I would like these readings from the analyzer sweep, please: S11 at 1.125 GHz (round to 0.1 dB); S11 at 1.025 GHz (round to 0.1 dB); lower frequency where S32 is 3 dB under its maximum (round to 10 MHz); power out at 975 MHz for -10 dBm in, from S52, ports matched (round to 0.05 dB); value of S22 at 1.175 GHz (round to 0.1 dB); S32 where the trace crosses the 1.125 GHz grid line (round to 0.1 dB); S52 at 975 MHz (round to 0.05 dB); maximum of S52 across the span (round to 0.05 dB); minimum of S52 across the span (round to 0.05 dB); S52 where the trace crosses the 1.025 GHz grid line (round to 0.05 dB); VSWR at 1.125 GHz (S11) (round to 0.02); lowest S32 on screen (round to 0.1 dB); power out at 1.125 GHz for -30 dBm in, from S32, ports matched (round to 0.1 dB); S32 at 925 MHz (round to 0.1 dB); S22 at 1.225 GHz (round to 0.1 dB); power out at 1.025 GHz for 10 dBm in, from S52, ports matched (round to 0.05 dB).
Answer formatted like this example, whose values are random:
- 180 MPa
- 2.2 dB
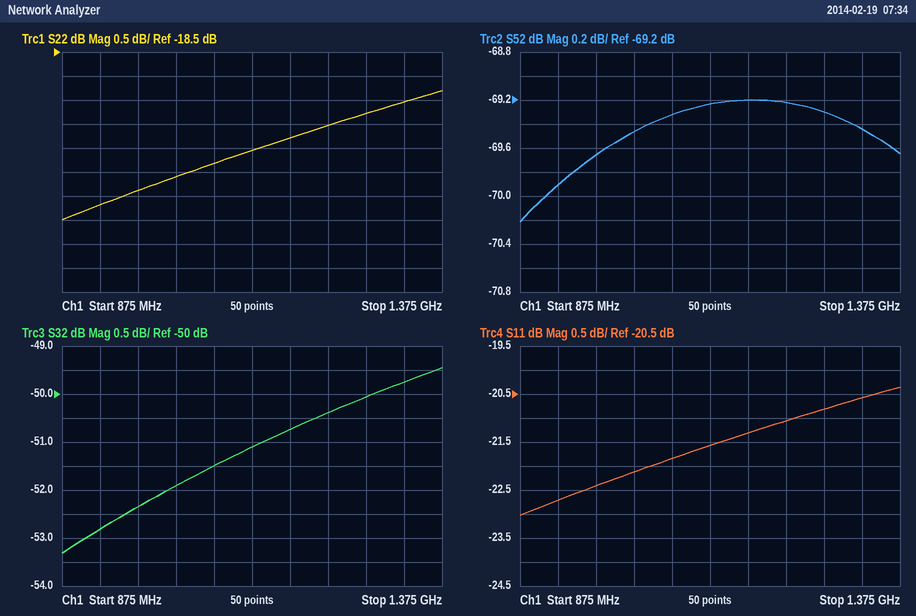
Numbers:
- -21.6 dB
- -22.1 dB
- 960 MHz
- -79.65 dBm
- -20.3 dB
- -51.1 dB
- -69.65 dB
- -69.20 dB
- -70.20 dB
- -69.45 dB
- 1.18
- -53.3 dB
- -81.1 dBm
- -52.8 dB
- -20.0 dB
- -59.45 dBm
